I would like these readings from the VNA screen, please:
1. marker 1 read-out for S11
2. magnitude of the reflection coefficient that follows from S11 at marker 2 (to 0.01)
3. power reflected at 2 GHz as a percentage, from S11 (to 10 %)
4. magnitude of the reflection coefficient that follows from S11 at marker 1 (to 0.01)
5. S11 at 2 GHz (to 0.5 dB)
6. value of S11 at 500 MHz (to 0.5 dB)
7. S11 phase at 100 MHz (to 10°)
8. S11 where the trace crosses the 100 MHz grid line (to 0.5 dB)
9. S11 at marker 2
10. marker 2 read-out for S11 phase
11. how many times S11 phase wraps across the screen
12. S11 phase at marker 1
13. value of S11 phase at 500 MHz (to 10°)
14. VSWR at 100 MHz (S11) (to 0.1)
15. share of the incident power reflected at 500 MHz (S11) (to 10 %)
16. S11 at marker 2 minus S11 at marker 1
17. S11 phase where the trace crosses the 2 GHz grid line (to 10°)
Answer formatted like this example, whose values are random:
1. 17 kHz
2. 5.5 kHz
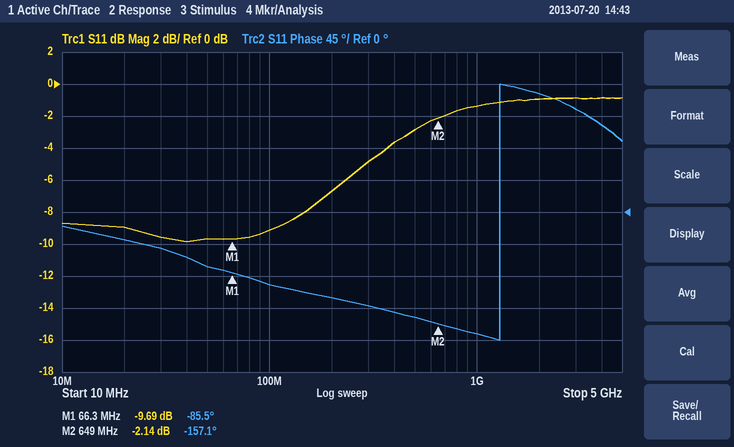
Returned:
1. -9.69 dB
2. 0.78
3. 80 %
4. 0.33
5. -1.0 dB
6. -3.0 dB
7. -100°
8. -9.0 dB
9. -2.14 dB
10. -157.1°
11. 1
12. -85.5°
13. -150°
14. 2.1
15. 50 %
16. 7.55 dB
17. 170°
